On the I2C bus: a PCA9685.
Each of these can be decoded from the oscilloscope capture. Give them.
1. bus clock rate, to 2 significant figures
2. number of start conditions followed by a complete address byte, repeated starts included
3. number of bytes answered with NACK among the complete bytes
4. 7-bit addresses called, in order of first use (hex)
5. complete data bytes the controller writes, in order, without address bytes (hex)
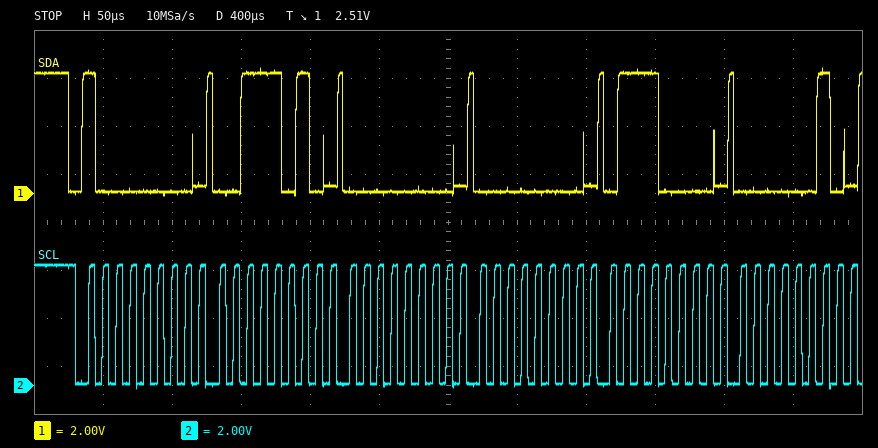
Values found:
100 kHz
1
0
0x40
3A 00 00 70 02
